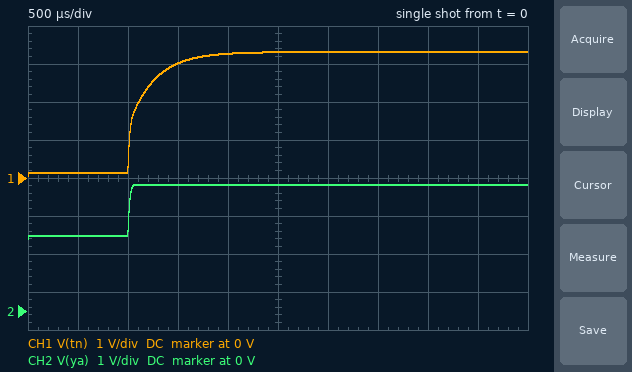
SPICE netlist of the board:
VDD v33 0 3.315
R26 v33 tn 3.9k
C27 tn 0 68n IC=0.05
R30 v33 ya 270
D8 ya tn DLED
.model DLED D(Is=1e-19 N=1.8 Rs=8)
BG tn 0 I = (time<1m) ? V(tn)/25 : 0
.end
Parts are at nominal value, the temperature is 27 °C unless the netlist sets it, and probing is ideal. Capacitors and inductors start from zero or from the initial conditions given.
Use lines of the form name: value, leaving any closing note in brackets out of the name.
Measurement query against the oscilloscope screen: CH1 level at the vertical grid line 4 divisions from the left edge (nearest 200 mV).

CH1 level at the vertical grid line 4 divisions from the left edge: 3.2 V
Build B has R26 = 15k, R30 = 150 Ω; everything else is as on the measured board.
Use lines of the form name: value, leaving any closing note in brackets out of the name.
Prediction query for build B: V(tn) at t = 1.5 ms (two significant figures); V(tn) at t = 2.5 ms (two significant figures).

V(tn) at t = 1.5 ms: 2.3 V
V(tn) at t = 2.5 ms: 2.9 V
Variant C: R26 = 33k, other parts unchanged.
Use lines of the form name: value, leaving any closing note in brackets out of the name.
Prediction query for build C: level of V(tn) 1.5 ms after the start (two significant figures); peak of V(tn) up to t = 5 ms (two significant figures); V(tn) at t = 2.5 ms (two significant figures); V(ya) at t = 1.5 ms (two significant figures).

level of V(tn) 1.5 ms after the start: 2.0 V
peak of V(tn) up to t = 5 ms: 3.0 V
V(tn) at t = 2.5 ms: 2.5 V
V(ya) at t = 1.5 ms: 3.3 V
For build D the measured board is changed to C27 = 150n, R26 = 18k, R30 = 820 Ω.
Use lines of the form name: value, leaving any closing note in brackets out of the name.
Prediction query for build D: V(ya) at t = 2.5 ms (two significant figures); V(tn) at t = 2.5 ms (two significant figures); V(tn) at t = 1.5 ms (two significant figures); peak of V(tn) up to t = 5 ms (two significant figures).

V(ya) at t = 2.5 ms: 3.3 V
V(tn) at t = 2.5 ms: 2.3 V
V(tn) at t = 1.5 ms: 1.8 V
peak of V(tn) up to t = 5 ms: 2.9 V
